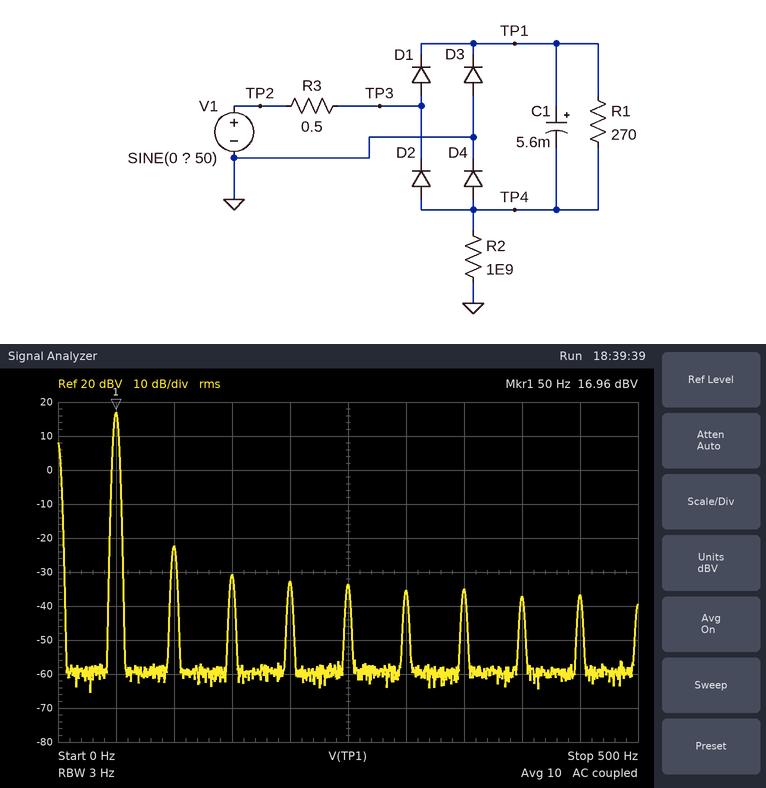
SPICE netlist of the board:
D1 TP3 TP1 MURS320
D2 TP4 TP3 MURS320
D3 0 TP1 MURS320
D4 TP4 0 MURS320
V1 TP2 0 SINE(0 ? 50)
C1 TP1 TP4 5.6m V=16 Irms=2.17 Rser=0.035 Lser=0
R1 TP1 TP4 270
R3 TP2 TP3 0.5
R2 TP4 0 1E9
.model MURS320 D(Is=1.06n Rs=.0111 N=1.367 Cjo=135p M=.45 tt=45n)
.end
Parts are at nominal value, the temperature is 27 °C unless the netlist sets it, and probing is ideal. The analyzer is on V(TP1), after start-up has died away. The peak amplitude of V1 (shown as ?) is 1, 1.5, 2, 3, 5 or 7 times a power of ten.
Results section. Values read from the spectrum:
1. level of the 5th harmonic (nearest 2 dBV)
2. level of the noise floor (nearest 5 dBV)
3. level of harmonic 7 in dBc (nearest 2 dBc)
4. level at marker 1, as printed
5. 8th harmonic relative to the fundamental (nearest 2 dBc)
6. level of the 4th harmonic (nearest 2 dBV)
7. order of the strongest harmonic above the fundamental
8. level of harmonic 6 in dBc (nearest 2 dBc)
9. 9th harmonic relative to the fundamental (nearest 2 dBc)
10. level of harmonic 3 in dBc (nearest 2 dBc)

-34 dBV
-60 dBV
-52 dBc
16.96 dBV
-54 dBc
-32 dBV
2
-52 dBc
-54 dBc
-48 dBc
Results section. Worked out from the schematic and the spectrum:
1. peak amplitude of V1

20 V
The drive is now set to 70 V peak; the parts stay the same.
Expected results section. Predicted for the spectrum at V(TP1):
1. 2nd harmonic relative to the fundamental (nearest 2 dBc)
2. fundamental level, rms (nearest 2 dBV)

-34 dBc
28 dBV
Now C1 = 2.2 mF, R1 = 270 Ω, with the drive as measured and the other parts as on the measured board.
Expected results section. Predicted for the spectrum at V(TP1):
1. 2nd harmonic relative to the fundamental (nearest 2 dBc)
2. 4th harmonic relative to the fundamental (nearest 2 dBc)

-40 dBc
-48 dBc
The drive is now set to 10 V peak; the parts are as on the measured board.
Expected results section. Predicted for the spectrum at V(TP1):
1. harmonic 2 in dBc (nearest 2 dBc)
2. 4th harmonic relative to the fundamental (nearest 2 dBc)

-44 dBc
-52 dBc
